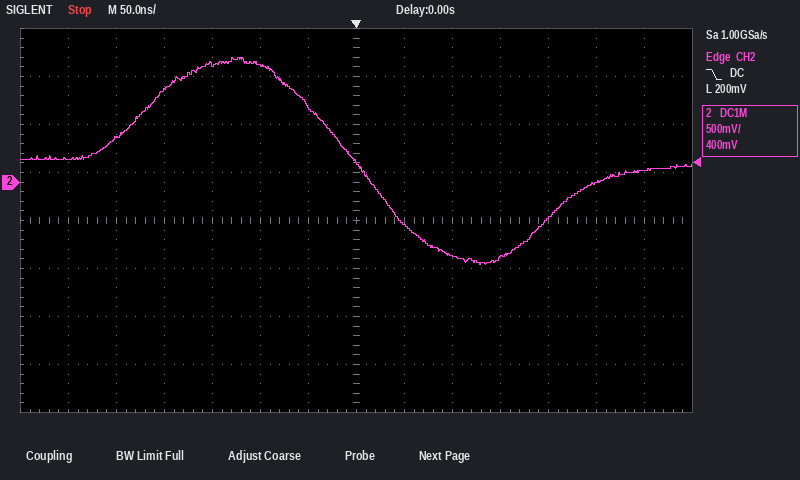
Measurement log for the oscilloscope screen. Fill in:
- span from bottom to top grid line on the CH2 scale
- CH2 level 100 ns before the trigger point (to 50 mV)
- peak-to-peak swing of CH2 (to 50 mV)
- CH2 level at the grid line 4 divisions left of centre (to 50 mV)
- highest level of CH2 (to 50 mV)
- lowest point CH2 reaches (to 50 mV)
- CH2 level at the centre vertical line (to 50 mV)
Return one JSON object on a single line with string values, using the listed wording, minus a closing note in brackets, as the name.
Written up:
{"span from bottom to top grid line on the CH2 scale": "4 V", "CH2 level 100 ns before the trigger point": "1.20 V", "peak-to-peak swing of CH2": "2.15 V", "CH2 level at the grid line 4 divisions left of centre": "950 mV", "highest level of CH2": "1.30 V", "lowest point CH2 reaches": "-850 mV", "CH2 level at the centre vertical line": "200 mV"}
